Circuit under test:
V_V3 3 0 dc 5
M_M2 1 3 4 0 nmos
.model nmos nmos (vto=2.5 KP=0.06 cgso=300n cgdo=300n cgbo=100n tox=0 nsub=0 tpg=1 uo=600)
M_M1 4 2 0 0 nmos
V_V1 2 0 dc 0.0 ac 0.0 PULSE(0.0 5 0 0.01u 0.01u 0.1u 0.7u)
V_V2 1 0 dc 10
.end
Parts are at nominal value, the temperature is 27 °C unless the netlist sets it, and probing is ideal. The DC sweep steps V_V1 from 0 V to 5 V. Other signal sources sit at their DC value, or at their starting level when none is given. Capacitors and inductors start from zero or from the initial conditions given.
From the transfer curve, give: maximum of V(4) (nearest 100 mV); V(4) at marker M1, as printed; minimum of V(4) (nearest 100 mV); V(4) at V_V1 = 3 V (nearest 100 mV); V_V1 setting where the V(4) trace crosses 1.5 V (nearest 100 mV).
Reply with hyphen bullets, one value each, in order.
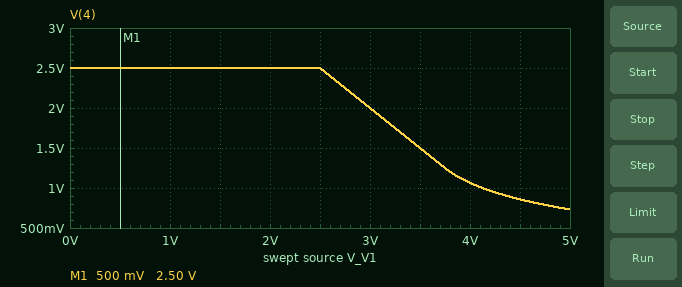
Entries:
- 2.5 V
- 2.50 V
- 700 mV
- 2.0 V
- 3.5 V
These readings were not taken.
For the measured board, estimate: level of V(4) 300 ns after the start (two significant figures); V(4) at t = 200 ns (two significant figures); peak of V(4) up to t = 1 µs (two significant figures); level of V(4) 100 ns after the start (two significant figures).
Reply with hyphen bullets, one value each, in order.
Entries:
- 2.5 V
- 2.5 V
- 4.0 V
- 730 mV
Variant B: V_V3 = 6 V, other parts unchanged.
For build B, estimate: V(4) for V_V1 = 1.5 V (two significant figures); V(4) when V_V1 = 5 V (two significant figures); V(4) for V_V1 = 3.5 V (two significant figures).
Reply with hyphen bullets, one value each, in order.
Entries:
- 3.5 V
- 1.3 V
- 2.5 V
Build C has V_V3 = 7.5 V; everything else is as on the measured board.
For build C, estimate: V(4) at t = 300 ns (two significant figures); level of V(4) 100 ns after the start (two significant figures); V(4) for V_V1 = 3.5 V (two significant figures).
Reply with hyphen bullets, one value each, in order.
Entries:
- 5.0 V
- 2.5 V
- 4.0 V
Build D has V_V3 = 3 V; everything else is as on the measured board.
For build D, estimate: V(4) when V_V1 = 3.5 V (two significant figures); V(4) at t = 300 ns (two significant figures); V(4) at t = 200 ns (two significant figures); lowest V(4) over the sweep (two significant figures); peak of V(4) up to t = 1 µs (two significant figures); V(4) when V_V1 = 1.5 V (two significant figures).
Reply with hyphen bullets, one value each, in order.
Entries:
- 89 mV
- 490 mV
- 480 mV
- 42 mV
- 3.0 V
- 500 mV
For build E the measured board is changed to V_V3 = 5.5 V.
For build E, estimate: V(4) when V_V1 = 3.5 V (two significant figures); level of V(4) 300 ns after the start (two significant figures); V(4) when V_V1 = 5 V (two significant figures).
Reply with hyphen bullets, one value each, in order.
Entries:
- 2.0 V
- 3.0 V
- 1.0 V
